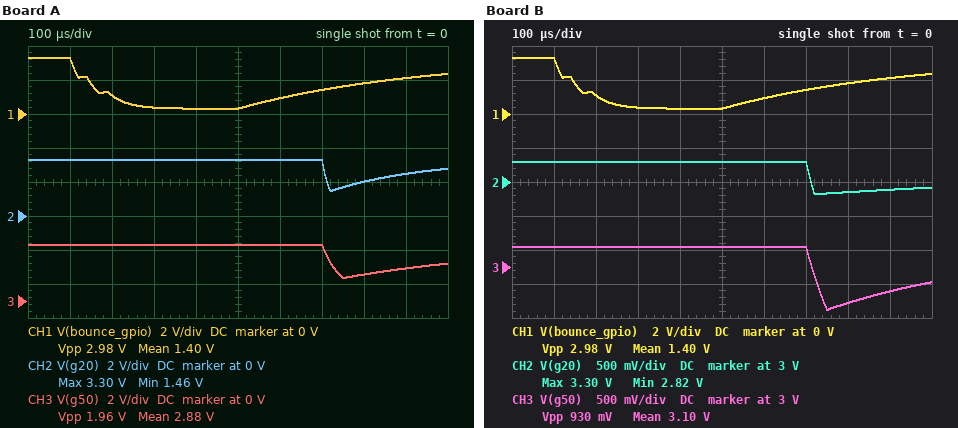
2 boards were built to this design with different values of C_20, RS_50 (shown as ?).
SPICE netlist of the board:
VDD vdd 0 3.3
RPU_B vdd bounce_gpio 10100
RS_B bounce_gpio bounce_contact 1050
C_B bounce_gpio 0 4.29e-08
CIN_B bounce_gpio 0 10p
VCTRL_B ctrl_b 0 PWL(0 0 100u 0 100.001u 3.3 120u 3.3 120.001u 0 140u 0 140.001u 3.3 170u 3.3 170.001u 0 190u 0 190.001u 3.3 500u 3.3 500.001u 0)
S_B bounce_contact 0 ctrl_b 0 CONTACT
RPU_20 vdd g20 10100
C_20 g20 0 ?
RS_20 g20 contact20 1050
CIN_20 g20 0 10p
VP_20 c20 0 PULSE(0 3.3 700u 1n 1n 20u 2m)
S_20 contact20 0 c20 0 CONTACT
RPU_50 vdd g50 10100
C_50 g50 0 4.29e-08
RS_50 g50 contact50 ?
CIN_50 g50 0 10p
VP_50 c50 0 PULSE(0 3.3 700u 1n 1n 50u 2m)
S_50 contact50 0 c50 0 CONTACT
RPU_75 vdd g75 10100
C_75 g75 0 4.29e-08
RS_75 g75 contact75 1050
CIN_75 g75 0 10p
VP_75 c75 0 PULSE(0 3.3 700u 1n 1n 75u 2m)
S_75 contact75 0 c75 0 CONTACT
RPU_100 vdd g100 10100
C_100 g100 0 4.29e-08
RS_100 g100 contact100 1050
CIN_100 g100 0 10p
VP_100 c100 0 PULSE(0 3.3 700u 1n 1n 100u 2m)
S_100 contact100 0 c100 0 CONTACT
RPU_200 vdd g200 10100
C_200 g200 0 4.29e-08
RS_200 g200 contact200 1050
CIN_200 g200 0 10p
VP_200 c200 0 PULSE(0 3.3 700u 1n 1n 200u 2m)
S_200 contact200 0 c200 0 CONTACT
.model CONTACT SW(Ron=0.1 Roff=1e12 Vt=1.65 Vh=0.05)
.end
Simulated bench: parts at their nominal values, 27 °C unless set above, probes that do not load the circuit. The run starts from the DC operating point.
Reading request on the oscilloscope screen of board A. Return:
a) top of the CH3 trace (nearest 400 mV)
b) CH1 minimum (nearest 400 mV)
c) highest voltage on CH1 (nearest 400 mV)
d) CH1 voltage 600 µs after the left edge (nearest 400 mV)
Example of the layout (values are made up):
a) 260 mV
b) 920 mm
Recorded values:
a) 3.2 V
b) 400 mV
c) 3.2 V
d) 800 mV
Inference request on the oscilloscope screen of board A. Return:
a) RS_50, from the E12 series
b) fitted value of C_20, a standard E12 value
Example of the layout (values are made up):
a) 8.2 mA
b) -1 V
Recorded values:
a) 1.2 kΩ
b) 22 nF
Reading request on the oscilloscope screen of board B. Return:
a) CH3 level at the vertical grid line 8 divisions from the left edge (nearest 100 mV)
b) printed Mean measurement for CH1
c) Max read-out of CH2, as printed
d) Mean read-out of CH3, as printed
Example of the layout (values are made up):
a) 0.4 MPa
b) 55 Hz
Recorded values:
a) 2.5 V
b) 1.40 V
c) 3.30 V
d) 3.10 V
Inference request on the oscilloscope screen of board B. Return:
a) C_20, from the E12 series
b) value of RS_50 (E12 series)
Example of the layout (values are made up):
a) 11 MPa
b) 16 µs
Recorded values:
a) 120 nF
b) 3.3 kΩ
